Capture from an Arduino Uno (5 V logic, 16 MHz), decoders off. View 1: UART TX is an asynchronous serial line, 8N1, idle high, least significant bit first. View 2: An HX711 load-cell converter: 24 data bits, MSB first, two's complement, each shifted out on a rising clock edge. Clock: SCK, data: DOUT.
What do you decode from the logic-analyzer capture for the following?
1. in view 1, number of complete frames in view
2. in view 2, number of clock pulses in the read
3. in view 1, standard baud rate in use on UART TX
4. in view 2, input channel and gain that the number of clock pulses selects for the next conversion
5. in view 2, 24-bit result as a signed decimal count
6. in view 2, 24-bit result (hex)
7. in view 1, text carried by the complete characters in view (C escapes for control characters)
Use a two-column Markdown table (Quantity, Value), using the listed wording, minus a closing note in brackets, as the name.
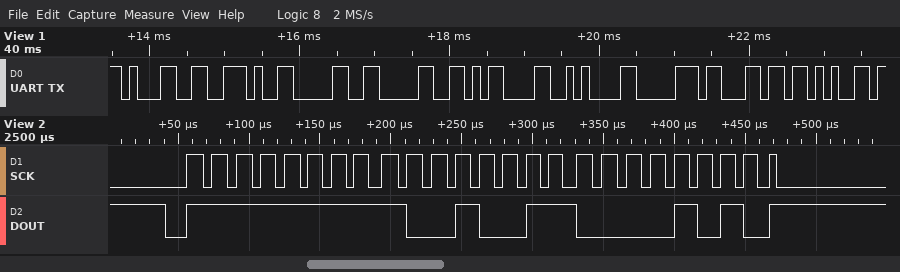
| Quantity | Value |
|---|---|
| in view 1, number of complete frames in view | 9 |
| in view 2, number of clock pulses in the read | 25 |
| in view 1, standard baud rate in use on UART TX | 9600 baud |
| in view 2, input channel and gain that the number of clock pulses selects for the next conversion | channel A, gain 128 |
| in view 2, 24-bit result as a signed decimal count | -27894 |
| in view 2, 24-bit result | 0xFF930A |
| in view 1, text carried by the complete characters in view | "1.00\r\nple" |
